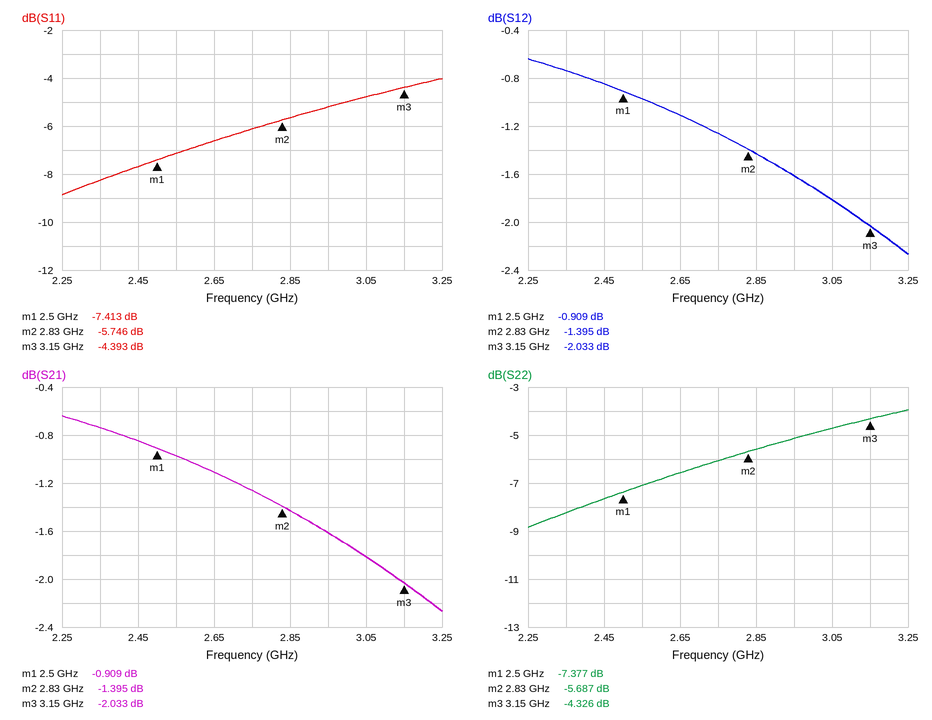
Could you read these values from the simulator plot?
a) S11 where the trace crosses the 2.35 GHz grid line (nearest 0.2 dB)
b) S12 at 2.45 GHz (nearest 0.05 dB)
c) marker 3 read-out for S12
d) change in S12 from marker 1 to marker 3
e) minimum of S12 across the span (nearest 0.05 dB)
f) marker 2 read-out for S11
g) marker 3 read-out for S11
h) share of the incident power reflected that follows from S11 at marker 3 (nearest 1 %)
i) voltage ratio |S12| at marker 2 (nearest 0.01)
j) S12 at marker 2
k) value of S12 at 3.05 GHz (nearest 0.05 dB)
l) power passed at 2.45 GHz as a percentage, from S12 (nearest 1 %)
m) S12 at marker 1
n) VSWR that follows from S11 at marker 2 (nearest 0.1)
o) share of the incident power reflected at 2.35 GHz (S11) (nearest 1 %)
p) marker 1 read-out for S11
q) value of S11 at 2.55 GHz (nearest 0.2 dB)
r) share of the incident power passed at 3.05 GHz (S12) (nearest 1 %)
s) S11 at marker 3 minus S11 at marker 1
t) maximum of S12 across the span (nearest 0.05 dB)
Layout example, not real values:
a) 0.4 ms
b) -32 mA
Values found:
a) -8.2 dB
b) -0.85 dB
c) -2.033 dB
d) -1.124 dB
e) -2.25 dB
f) -5.746 dB
g) -4.393 dB
h) 36 %
i) 0.85
j) -1.395 dB
k) -1.80 dB
l) 82 %
m) -0.909 dB
n) 3.1
o) 15 %
p) -7.413 dB
q) -7.2 dB
r) 66 %
s) 3.020 dB
t) -0.65 dB
